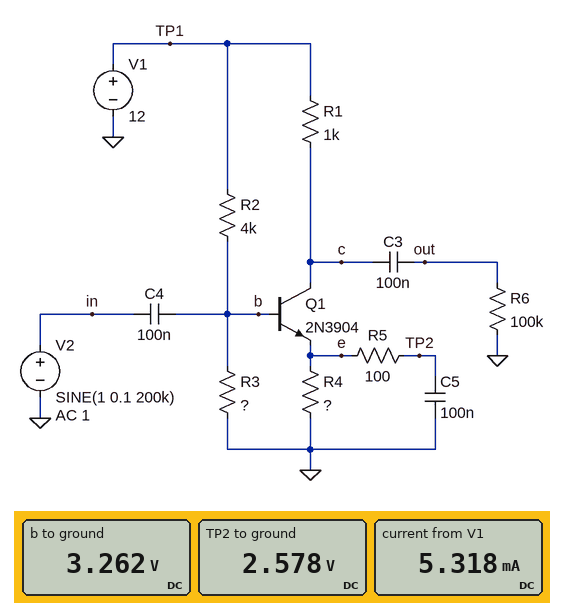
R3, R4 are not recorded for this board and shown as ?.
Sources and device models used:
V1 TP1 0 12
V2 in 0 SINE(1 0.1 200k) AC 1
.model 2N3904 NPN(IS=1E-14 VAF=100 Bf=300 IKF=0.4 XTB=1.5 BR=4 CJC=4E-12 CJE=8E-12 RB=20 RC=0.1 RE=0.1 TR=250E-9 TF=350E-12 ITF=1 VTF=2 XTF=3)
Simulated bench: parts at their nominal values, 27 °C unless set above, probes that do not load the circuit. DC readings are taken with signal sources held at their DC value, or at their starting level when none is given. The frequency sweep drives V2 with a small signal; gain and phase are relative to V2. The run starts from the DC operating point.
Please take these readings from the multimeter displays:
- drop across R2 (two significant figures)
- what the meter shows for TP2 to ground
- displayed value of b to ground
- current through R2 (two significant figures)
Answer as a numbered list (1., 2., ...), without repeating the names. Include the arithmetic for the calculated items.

1. 12 V - 3.262 V = 8.7 V
2. 2.578 V
3. 3.262 V
4. (12 V - 3.262 V) / 4 kΩ = 2.2 mA
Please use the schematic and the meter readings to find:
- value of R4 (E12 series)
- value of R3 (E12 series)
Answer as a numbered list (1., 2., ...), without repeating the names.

1. 820 Ω
2. 1.5 kΩ
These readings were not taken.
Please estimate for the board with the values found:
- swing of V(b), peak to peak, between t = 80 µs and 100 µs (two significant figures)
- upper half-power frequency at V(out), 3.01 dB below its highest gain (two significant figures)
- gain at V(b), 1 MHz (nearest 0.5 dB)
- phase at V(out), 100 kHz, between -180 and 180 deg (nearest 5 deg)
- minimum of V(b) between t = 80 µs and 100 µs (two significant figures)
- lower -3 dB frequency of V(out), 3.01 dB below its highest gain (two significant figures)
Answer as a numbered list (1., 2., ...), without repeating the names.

1. 200 mV
2. 64 MHz
3. 0 dB
4. -170 deg
5. 3.2 V
6. 15 kHz
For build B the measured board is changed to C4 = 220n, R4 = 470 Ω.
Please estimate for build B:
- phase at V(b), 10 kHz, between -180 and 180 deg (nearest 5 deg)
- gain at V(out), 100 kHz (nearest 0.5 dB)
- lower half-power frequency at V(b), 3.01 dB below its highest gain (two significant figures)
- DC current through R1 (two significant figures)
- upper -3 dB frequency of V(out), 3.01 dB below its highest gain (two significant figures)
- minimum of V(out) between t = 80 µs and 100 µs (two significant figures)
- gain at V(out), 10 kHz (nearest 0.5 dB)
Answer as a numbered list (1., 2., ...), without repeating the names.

1. 5 deg
2. 21.0 dB
3. 670 Hz
4. 5.4 mA
5. 55 MHz
6. -1.1 V
7. 16.0 dB
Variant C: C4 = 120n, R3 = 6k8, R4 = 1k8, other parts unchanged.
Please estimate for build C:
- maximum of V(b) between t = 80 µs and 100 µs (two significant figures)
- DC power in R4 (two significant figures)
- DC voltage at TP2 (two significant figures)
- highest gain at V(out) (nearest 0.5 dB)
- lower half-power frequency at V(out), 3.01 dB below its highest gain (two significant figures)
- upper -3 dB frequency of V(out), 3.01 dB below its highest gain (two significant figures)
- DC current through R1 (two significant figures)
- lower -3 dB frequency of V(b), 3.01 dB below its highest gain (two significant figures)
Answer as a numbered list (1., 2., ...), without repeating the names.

1. 7.6 V
2. 26 mW
3. 6.8 V
4. 19.5 dB
5. 15 kHz
6. 41 MHz
7. 3.8 mA
8. 530 Hz
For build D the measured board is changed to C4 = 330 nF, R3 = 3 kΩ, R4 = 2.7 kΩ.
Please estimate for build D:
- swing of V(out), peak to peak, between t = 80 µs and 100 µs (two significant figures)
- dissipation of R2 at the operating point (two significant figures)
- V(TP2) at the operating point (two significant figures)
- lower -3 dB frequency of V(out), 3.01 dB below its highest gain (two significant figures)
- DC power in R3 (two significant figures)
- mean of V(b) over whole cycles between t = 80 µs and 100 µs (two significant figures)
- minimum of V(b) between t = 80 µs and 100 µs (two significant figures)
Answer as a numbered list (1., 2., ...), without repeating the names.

1. 1.7 V
2. 12 mW
3. 4.5 V
4. 14 kHz
5. 8.8 mW
6. 5.1 V
7. 5.0 V
